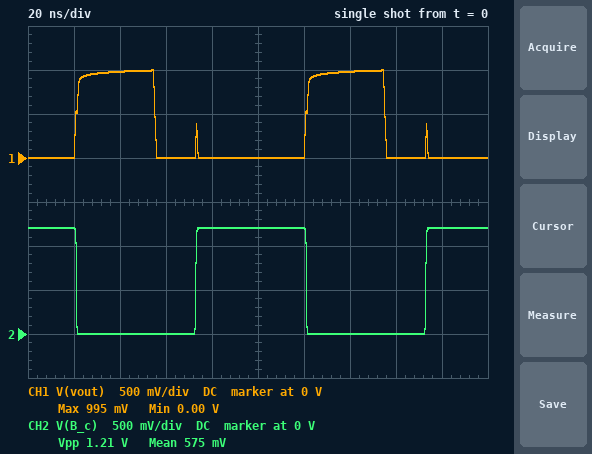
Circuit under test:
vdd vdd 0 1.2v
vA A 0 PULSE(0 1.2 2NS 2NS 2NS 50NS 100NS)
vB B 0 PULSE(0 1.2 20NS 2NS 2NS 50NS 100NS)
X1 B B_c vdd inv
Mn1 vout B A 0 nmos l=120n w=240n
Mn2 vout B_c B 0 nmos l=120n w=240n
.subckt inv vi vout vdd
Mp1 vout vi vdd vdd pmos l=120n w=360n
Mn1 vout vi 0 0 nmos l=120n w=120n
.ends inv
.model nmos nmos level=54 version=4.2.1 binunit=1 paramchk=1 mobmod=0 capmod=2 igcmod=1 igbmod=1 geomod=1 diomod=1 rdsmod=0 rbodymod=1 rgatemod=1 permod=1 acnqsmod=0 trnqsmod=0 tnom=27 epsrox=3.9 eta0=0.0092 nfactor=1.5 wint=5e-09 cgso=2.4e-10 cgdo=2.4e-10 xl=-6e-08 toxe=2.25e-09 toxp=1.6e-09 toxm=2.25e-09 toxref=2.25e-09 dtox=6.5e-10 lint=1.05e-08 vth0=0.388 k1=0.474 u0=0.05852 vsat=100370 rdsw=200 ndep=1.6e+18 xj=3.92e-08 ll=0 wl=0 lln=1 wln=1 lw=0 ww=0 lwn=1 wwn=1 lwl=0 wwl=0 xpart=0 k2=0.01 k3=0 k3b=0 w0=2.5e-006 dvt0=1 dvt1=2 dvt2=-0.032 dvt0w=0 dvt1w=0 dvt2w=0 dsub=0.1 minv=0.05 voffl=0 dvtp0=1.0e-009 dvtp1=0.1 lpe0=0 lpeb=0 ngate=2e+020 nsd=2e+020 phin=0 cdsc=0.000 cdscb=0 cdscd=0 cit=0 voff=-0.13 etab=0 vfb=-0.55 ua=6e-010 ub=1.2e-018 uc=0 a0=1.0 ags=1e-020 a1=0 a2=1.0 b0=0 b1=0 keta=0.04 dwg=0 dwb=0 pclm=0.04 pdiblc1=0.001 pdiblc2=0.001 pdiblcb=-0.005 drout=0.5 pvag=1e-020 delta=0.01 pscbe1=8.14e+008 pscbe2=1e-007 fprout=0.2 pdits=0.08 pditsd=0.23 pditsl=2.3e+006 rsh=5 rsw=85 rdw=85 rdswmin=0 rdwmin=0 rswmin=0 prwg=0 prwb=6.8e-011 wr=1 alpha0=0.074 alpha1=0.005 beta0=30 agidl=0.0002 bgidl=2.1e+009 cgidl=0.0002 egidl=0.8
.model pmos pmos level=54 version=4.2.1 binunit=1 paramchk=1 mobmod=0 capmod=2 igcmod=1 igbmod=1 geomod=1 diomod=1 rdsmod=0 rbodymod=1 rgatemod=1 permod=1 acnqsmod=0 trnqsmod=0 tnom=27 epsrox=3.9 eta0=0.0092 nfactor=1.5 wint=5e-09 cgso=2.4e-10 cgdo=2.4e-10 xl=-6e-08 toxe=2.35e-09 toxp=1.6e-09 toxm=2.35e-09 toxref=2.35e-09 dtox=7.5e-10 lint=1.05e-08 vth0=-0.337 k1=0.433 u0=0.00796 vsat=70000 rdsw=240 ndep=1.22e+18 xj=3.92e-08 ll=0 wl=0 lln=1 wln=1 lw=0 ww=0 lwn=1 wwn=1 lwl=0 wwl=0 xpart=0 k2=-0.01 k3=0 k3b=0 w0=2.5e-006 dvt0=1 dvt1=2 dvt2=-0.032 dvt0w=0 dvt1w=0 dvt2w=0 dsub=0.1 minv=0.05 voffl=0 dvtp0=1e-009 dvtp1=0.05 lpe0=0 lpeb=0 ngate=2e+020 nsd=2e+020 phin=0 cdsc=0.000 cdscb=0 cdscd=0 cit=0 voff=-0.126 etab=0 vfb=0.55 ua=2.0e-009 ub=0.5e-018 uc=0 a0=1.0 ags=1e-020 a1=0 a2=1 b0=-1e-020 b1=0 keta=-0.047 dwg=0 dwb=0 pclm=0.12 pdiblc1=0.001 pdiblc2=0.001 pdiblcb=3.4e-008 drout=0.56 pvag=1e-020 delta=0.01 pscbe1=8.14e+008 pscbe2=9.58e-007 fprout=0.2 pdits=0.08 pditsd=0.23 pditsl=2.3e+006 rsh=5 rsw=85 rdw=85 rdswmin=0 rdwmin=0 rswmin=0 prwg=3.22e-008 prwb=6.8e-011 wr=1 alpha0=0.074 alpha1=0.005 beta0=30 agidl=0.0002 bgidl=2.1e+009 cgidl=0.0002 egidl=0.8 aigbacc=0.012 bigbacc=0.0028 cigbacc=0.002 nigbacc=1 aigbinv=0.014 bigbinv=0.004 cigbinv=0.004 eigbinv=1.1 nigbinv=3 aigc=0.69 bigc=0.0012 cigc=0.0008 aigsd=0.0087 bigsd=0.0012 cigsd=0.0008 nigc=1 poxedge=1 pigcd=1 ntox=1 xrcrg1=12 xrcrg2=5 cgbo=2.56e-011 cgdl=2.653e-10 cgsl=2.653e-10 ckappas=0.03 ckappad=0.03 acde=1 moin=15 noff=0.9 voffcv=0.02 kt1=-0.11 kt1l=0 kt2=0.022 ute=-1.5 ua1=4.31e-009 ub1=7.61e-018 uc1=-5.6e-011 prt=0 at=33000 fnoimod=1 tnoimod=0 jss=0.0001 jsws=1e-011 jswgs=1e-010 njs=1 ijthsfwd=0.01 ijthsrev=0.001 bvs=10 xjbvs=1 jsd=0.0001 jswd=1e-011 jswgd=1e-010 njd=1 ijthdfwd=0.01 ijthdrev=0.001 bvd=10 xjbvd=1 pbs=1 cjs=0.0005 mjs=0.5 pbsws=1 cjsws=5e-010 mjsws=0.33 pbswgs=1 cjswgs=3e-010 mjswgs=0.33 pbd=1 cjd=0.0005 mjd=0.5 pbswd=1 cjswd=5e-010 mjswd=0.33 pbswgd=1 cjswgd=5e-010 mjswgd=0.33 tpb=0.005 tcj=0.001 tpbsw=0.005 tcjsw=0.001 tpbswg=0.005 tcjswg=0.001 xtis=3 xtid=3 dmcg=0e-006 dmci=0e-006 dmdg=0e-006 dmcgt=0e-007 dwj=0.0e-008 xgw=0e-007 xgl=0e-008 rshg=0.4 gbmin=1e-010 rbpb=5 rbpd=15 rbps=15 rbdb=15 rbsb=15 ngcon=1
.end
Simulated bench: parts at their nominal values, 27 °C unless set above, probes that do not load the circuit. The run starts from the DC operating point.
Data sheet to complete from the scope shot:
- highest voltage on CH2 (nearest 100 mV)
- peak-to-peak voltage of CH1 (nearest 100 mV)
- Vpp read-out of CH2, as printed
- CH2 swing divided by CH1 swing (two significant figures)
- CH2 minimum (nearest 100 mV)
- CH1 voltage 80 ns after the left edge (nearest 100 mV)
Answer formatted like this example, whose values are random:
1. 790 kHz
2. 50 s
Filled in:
1. 1.2 V
2. 1.0 V
3. 1.21 V
4. 1.2
5. 0 V
6. 0 V
